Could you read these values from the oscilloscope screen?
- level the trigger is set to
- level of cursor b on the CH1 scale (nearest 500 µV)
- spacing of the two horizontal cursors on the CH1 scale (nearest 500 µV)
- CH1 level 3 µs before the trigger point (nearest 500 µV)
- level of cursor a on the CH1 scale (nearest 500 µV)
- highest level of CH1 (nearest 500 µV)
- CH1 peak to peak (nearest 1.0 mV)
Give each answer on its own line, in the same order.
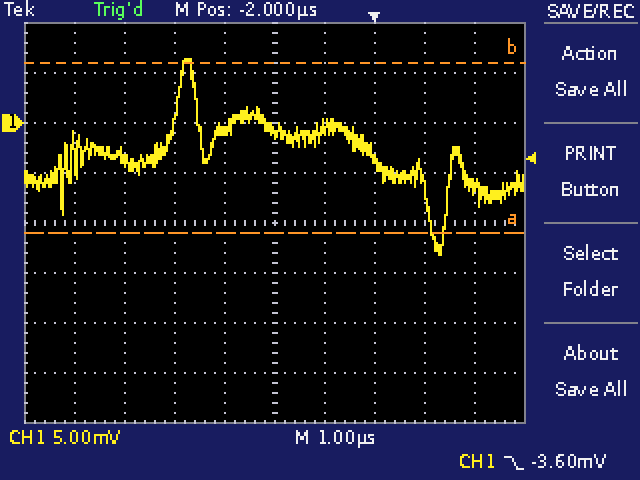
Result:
-3.60 mV
6.0 mV
17.0 mV
-1.0 mV
-11.0 mV
6.5 mV
20.0 mV
